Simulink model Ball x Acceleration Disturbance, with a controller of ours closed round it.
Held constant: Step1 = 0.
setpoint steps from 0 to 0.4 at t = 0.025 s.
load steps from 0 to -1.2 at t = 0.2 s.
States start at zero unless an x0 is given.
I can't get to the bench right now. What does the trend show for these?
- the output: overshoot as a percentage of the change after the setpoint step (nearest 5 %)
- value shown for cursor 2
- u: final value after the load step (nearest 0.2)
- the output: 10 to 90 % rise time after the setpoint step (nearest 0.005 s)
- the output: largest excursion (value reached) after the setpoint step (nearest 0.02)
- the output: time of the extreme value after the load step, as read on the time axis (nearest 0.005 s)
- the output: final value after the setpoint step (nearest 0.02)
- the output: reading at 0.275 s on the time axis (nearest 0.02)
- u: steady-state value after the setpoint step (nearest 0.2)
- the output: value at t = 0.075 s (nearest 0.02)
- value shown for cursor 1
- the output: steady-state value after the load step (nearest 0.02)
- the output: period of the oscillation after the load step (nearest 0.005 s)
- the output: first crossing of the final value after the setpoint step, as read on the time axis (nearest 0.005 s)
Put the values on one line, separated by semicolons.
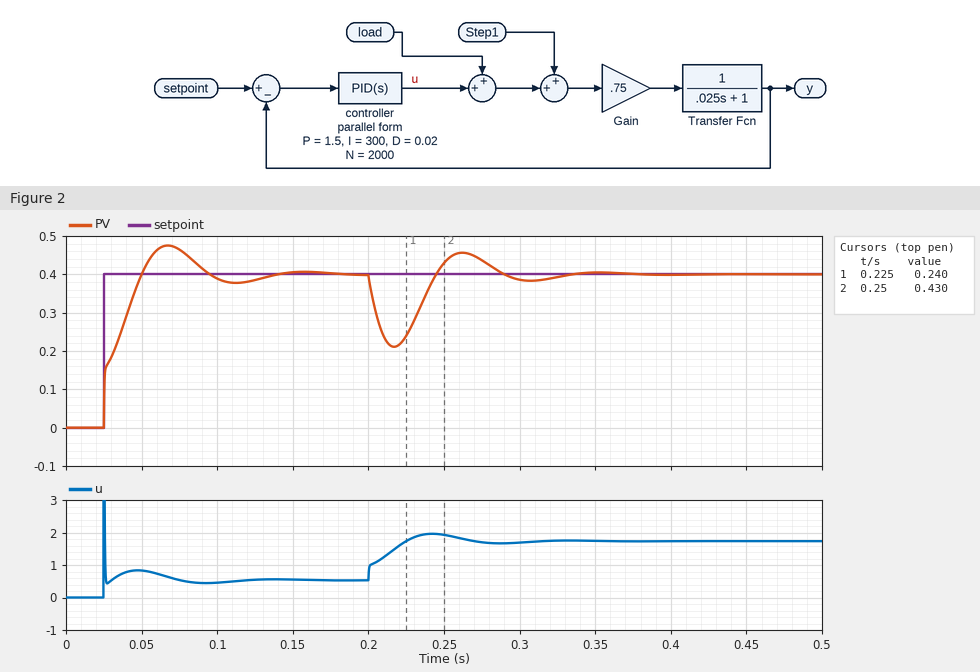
20 %; 0.430; 1.8; 0.020 s; 0.48; 0.215 s; 0.40; 0.44; 0.6; 0.46; 0.240; 0.40; 0.090 s; 0.050 s
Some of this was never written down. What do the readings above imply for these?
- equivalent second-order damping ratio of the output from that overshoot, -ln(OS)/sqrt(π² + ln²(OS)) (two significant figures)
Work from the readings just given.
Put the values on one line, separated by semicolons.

0.46
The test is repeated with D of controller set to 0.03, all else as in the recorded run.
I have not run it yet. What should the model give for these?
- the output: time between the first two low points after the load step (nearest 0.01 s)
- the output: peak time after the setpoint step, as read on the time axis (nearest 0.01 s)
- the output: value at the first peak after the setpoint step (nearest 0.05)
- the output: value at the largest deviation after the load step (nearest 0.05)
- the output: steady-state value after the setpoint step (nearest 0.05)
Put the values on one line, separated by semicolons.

0.10 s; 0.07 s; 0.45; 0.20; 0.40
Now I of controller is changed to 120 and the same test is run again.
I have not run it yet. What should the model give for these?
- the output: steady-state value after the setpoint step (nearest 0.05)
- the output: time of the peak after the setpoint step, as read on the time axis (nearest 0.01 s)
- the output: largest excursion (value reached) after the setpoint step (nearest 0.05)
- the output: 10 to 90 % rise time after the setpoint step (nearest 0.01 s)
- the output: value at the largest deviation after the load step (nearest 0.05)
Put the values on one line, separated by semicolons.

0.40; 0.10 s; 0.45; 0.04 s; 0.15
